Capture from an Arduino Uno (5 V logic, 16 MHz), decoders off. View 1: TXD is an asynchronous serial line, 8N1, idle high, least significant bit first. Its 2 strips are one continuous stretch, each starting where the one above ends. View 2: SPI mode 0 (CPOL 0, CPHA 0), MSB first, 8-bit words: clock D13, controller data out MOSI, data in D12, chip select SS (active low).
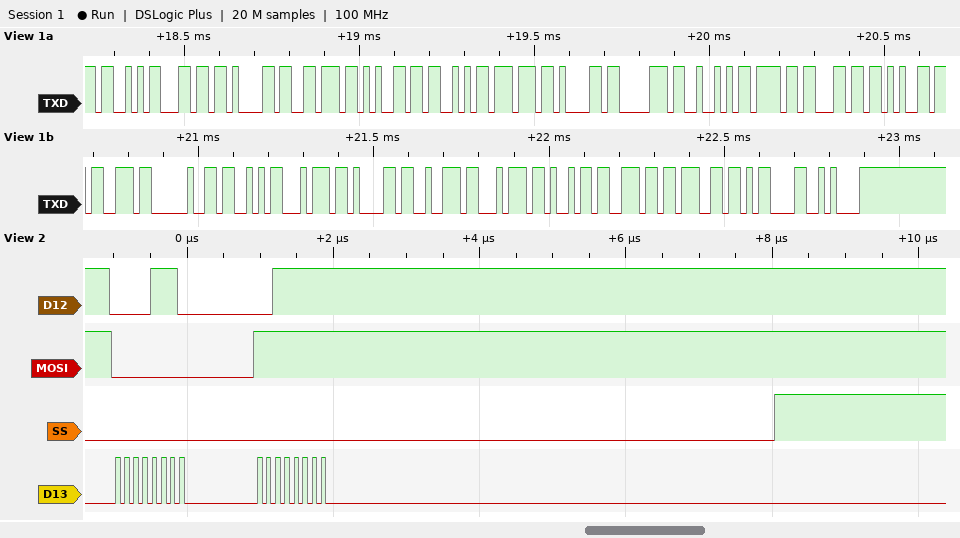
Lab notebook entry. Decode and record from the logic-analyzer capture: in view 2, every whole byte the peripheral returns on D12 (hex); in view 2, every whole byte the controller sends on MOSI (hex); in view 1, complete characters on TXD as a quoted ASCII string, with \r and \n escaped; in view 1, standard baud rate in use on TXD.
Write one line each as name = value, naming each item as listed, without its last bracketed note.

in view 2, every whole byte the peripheral returns on D12 = 0x0E 0x3F
in view 2, every whole byte the controller sends on MOSI = 0x00 0xFF
in view 1, complete characters on TXD as a quoted ASCII string, with \r and \n escaped = "SlaveSwapRoles Starting\r\n"
in view 1, standard baud rate in use on TXD = 57600 baud
